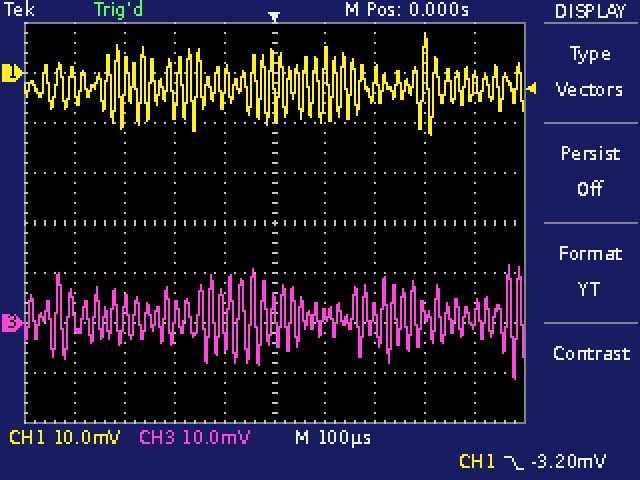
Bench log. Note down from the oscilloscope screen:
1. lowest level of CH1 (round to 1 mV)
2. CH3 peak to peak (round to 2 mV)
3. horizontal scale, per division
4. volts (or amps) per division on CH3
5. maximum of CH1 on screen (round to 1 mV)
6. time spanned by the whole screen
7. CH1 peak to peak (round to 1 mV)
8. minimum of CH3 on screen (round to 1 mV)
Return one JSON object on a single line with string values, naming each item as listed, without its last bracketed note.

{"lowest level of CH1": "-12 mV", "CH3 peak to peak": "22 mV", "horizontal scale, per division": "100 µs", "volts (or amps) per division on CH3": "10 mV", "maximum of CH1 on screen": "8 mV", "time spanned by the whole screen": "1 ms", "CH1 peak to peak": "20 mV", "minimum of CH3 on screen": "-11 mV"}
